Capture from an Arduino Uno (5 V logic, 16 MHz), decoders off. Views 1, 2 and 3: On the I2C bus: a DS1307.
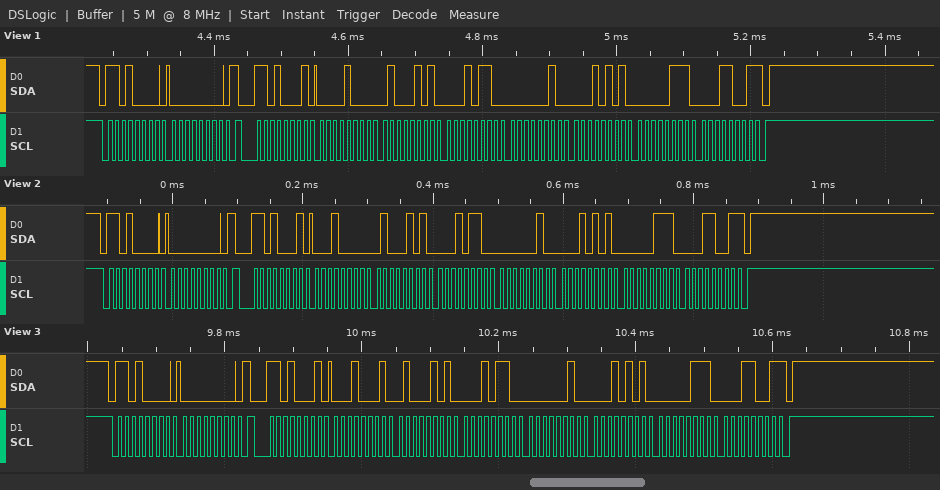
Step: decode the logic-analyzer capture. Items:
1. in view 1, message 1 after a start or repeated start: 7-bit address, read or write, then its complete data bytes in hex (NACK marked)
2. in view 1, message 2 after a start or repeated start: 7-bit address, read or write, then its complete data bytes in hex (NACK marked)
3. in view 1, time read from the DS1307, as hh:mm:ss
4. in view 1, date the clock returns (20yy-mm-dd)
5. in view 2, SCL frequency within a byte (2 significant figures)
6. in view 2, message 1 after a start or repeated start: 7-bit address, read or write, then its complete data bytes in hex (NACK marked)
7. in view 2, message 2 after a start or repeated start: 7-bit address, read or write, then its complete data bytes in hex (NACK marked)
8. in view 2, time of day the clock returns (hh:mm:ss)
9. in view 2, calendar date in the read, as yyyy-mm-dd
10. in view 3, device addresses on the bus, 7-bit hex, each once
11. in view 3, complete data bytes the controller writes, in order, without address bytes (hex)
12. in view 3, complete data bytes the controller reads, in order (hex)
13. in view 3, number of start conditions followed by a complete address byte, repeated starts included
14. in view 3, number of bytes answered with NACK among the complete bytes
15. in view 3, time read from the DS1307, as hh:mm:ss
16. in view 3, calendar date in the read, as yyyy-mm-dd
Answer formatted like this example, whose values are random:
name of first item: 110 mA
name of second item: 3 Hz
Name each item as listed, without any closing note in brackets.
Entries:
in view 1, message 1 after a start or repeated start: 7-bit address, read or write, then its complete data bytes in hex: 0x68 write: 00
in view 1, message 2 after a start or repeated start: 7-bit address, read or write, then its complete data bytes in hex: 0x68 read: 08 45 16 02 15 07 19 NACK
in view 1, time read from the DS1307, as hh:mm:ss: 16:45:08
in view 1, date the clock returns: 2019-07-15
in view 2, SCL frequency within a byte: 100 kHz
in view 2, message 1 after a start or repeated start: 7-bit address, read or write, then its complete data bytes in hex: 0x68 write: 00
in view 2, message 2 after a start or repeated start: 7-bit address, read or write, then its complete data bytes in hex: 0x68 read: 10 45 16 02 15 07 19 NACK
in view 2, time of day the clock returns: 16:45:10
in view 2, calendar date in the read, as yyyy-mm-dd: 2019-07-15
in view 3, device addresses on the bus, 7-bit hex, each once: 0x68
in view 3, complete data bytes the controller writes, in order, without address bytes: 00
in view 3, complete data bytes the controller reads, in order: 11 45 16 02 15 07 19
in view 3, number of start conditions followed by a complete address byte, repeated starts included: 2
in view 3, number of bytes answered with NACK among the complete bytes: 1
in view 3, time read from the DS1307, as hh:mm:ss: 16:45:11
in view 3, calendar date in the read, as yyyy-mm-dd: 2019-07-15
